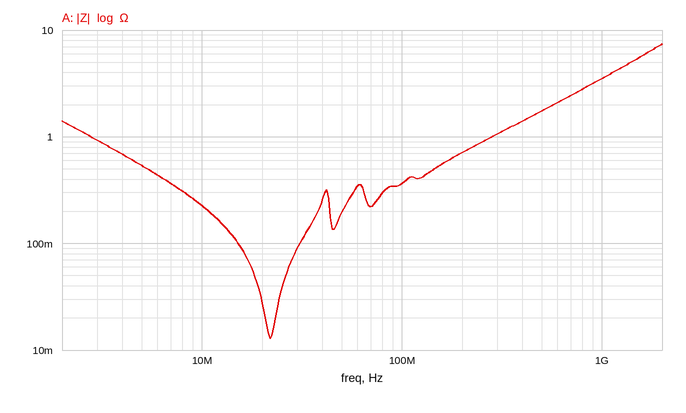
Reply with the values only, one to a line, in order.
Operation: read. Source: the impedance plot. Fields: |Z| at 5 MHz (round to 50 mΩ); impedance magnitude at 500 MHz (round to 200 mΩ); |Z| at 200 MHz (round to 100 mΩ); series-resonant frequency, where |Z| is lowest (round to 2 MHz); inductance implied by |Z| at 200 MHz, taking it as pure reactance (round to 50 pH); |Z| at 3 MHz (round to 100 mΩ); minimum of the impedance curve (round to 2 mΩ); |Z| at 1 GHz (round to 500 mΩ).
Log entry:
550 mΩ
1.8 Ω
700 mΩ
22 MHz
550 pH
900 mΩ
12 mΩ
3.5 Ω
